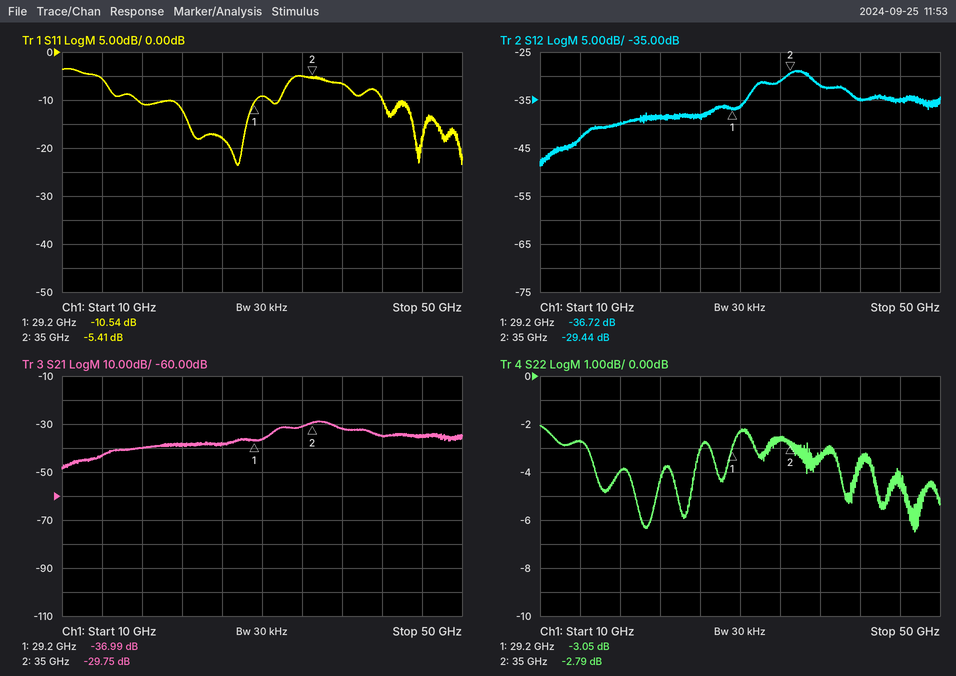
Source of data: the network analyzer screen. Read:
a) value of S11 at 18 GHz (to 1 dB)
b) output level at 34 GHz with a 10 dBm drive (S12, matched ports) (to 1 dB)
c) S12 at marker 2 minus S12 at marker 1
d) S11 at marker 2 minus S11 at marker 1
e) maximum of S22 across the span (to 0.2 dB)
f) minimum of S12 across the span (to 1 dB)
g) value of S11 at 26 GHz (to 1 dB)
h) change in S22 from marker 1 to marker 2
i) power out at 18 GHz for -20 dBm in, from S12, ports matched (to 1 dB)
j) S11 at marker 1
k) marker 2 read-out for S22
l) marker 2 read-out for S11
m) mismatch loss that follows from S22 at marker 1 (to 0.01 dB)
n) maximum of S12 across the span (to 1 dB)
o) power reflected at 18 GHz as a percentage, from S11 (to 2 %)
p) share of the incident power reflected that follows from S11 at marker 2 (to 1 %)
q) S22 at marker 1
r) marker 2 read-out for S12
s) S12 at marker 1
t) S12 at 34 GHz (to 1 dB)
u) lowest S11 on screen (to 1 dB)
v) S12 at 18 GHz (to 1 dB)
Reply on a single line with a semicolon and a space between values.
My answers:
-11 dB; -21 dBm; 7.28 dB; 5.13 dB; -2.0 dB; -49 dB; -18 dB; 0.26 dB; -60 dBm; -10.54 dB; -2.79 dB; -5.41 dB; 2.97 dB; -29 dB; 8 %; 29 %; -3.05 dB; -29.44 dB; -36.72 dB; -31 dB; -24 dB; -40 dB
